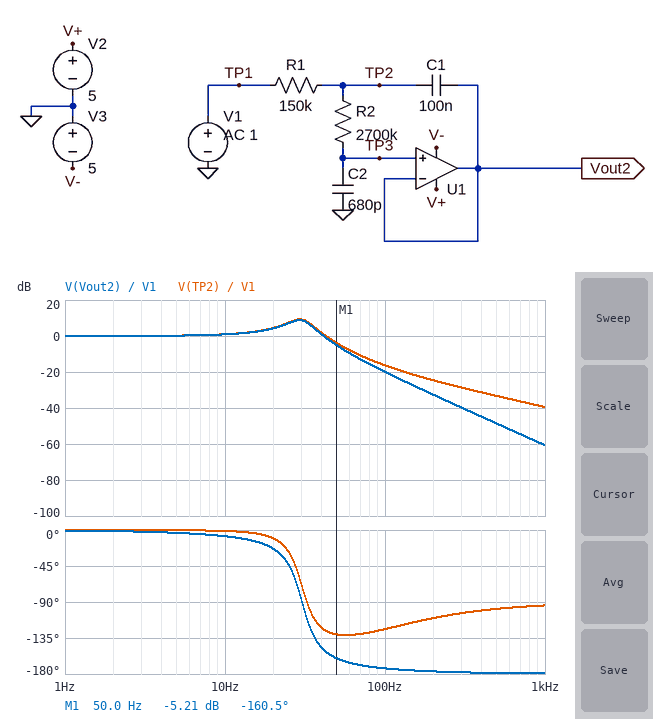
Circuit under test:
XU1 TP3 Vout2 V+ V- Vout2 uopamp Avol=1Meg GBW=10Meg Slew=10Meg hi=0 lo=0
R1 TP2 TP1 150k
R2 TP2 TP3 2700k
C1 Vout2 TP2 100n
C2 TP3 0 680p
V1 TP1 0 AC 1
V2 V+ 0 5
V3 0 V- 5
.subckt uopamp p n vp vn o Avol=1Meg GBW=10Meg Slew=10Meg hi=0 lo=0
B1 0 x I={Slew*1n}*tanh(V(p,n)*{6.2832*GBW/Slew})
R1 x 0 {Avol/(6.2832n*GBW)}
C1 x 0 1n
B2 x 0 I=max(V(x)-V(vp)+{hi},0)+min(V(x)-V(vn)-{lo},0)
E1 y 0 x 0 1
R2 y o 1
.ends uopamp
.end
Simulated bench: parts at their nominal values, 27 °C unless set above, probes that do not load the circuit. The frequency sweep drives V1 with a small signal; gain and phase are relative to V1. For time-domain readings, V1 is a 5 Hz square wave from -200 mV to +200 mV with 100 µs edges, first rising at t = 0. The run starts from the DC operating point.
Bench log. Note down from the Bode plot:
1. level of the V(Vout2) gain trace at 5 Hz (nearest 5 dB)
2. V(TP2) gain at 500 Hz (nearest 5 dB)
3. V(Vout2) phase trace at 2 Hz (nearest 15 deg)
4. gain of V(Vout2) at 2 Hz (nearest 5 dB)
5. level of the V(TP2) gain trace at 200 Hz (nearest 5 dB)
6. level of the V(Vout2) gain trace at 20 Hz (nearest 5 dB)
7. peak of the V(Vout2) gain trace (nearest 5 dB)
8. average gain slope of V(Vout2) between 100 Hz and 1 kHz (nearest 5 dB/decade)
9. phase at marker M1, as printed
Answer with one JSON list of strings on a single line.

["0 dB", "-35 dB", "0 deg", "0 dB", "-25 dB", "5 dB", "10 dB", "-40 dB/decade", "-160.5 deg"]
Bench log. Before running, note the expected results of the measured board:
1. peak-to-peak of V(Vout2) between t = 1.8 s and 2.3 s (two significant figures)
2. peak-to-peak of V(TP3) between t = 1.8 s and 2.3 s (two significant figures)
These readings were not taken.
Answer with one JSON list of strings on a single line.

["830 mV", "830 mV"]
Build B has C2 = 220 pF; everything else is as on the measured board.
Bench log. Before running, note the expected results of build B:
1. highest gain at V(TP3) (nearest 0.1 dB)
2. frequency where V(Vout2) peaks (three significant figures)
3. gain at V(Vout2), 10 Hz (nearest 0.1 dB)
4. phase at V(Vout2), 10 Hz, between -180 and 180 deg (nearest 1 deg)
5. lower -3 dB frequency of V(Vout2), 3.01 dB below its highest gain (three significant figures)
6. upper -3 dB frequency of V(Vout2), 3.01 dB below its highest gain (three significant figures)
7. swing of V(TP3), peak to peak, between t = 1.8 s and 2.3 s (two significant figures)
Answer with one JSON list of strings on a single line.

["13.6 dB", "52.7 Hz", "0.3 dB", "-2 deg", "46.8 Hz", "58.1 Hz", "980 mV"]
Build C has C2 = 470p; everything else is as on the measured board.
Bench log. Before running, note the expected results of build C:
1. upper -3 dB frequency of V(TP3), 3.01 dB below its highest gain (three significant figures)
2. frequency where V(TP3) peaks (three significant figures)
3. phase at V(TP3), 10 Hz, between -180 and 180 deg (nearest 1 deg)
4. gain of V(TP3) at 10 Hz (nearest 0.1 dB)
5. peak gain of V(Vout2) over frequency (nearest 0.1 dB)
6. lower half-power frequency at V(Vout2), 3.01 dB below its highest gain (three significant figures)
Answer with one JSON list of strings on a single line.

["40.9 Hz", "35.6 Hz", "-5 deg", "0.6 dB", "10.4 dB", "29.4 Hz"]
